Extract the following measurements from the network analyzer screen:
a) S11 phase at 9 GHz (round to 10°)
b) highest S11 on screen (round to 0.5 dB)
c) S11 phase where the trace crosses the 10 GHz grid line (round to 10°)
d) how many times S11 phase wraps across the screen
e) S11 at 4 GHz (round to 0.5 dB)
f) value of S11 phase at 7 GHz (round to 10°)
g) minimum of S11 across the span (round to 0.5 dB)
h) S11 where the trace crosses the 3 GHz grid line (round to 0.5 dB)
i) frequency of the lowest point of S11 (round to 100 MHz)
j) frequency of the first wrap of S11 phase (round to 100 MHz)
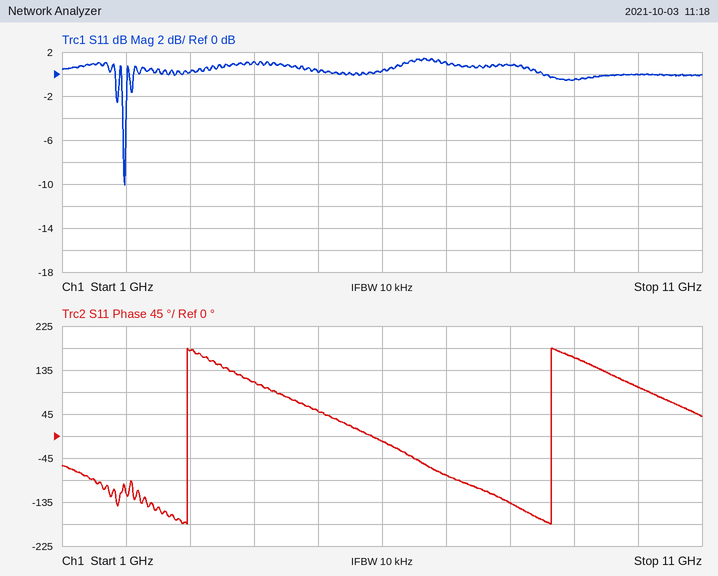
160°
1.5 dB
100°
2
1.0 dB
-80°
-10.0 dB
0.0 dB
2.0 GHz
3.0 GHz
